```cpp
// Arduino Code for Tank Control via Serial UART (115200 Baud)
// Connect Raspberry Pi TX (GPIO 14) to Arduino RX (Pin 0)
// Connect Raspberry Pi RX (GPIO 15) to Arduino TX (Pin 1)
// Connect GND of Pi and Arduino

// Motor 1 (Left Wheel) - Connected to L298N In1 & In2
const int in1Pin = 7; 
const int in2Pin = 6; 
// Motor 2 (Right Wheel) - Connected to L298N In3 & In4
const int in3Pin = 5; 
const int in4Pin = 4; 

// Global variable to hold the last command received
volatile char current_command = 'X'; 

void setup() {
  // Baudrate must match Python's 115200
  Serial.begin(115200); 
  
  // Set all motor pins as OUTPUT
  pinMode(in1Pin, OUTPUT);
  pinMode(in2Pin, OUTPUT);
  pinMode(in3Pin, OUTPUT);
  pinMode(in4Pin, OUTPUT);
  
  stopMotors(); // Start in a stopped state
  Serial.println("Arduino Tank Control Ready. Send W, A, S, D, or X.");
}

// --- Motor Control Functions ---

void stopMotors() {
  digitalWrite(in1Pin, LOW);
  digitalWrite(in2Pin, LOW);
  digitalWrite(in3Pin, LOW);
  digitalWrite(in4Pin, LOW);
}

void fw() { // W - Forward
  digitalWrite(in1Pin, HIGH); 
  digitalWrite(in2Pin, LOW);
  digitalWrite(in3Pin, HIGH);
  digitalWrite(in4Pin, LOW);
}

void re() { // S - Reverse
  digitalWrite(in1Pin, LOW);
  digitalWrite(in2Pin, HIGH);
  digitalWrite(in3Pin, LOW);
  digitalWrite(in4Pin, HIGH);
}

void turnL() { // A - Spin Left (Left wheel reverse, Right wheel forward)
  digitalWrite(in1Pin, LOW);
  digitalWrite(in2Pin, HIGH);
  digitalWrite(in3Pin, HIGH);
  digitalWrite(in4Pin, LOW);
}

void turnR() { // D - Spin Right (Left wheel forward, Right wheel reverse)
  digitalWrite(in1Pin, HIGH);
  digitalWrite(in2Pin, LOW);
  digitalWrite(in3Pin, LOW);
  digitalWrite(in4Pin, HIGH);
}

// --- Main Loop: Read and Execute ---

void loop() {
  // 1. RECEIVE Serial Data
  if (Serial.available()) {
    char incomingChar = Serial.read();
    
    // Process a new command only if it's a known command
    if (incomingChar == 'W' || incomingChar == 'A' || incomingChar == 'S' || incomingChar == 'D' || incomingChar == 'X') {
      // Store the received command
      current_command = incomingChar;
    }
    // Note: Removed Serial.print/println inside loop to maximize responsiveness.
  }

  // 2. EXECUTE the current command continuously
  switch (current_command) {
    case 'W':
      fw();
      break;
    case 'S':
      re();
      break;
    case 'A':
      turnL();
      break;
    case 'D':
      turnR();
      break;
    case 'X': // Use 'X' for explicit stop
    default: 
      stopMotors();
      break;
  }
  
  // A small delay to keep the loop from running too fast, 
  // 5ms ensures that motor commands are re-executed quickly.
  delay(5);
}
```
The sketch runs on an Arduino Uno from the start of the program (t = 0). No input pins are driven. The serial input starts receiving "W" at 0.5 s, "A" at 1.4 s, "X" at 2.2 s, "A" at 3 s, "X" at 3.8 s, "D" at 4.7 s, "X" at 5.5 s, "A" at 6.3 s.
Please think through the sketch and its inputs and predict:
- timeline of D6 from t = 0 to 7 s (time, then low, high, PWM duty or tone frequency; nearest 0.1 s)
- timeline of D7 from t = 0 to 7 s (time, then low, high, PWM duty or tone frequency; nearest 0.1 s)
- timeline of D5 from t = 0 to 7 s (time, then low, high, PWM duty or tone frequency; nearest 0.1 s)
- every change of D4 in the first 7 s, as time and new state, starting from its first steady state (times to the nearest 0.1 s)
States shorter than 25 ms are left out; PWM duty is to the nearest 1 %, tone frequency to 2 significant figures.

0 s low; 1.4 s high; 2.2 s low; 3 s high; 3.8 s low; 6.3 s high
0 s low; 0.5 s high; 1.4 s low; 4.7 s high; 5.5 s low
0 s low; 0.5 s high; 2.2 s low; 3 s high; 3.8 s low; 6.3 s high
0 s low; 4.7 s high; 5.5 s low
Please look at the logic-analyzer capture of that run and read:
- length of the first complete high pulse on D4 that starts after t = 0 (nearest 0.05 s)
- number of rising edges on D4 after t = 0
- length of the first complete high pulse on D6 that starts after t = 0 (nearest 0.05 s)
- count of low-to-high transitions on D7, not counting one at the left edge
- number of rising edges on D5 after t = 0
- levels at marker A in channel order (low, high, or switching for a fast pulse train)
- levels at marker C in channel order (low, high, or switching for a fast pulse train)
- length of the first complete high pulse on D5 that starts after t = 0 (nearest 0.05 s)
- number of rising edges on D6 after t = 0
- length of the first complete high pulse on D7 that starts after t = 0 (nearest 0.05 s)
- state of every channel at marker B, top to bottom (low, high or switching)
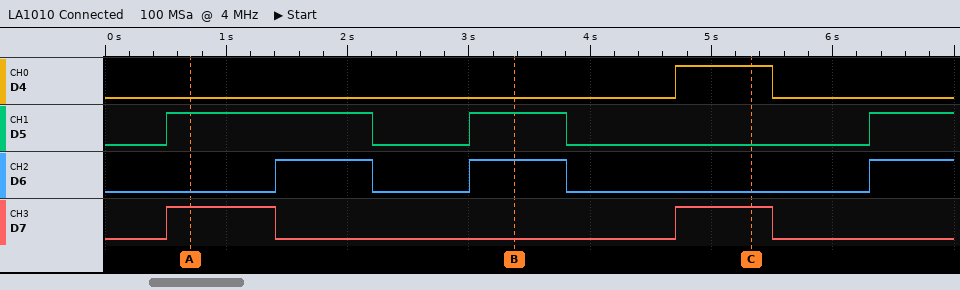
0.80 s
1
0.80 s
2
3
D4 low, D5 high, D6 low, D7 high
D4 high, D5 low, D6 low, D7 high
1.70 s
3
0.90 s
D4 low, D5 high, D6 high, D7 low
